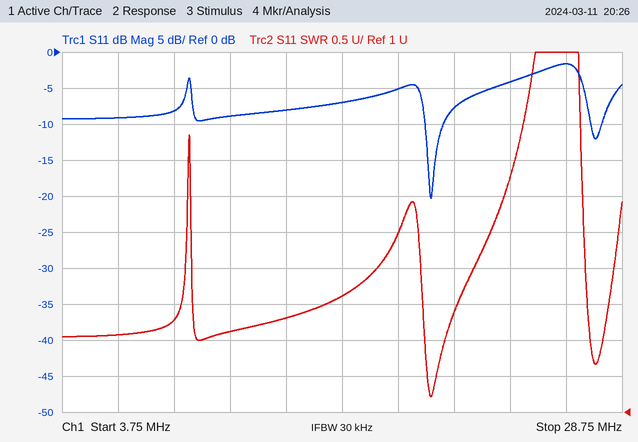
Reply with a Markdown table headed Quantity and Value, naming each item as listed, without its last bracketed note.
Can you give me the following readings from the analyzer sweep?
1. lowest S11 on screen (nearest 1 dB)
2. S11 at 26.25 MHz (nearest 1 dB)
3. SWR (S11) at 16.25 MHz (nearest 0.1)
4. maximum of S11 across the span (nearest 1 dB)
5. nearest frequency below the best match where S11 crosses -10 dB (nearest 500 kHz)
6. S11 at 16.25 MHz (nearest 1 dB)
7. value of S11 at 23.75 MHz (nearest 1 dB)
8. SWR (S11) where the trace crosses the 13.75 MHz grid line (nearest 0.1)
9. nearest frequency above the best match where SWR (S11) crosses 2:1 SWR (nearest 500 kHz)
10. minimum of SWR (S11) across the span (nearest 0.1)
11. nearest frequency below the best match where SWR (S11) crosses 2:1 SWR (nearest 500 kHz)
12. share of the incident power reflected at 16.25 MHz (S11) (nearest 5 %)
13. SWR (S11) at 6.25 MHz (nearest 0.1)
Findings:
| Quantity | Value |
|---|---|
| lowest S11 on screen | -20 dB |
| S11 at 26.25 MHz | -2 dB |
| SWR (S11) at 16.25 MHz | 2.6 |
| maximum of S11 across the span | -2 dB |
| nearest frequency below the best match where S11 crosses -10 dB | 20.0 MHz |
| S11 at 16.25 MHz | -7 dB |
| value of S11 at 23.75 MHz | -4 dB |
| SWR (S11) where the trace crosses the 13.75 MHz grid line | 2.3 |
| nearest frequency above the best match where SWR (S11) crosses 2:1 SWR | 21.0 MHz |
| minimum of SWR (S11) across the span | 1.2 |
| nearest frequency below the best match where SWR (S11) crosses 2:1 SWR | 20.0 MHz |
| share of the incident power reflected at 16.25 MHz (S11) | 20 % |
| SWR (S11) at 6.25 MHz | 2.1 |
